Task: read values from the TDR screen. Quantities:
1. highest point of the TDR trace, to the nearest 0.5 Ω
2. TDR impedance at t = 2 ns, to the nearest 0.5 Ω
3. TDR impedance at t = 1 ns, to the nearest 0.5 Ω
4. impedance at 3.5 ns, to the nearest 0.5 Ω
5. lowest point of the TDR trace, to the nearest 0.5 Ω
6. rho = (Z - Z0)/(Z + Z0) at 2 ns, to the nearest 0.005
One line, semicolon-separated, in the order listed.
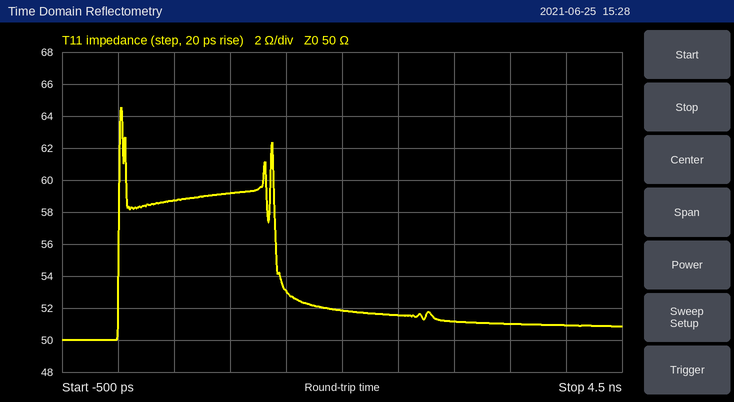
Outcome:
64.5 Ω; 52.0 Ω; 59.0 Ω; 51.0 Ω; 50.0 Ω; +0.020
